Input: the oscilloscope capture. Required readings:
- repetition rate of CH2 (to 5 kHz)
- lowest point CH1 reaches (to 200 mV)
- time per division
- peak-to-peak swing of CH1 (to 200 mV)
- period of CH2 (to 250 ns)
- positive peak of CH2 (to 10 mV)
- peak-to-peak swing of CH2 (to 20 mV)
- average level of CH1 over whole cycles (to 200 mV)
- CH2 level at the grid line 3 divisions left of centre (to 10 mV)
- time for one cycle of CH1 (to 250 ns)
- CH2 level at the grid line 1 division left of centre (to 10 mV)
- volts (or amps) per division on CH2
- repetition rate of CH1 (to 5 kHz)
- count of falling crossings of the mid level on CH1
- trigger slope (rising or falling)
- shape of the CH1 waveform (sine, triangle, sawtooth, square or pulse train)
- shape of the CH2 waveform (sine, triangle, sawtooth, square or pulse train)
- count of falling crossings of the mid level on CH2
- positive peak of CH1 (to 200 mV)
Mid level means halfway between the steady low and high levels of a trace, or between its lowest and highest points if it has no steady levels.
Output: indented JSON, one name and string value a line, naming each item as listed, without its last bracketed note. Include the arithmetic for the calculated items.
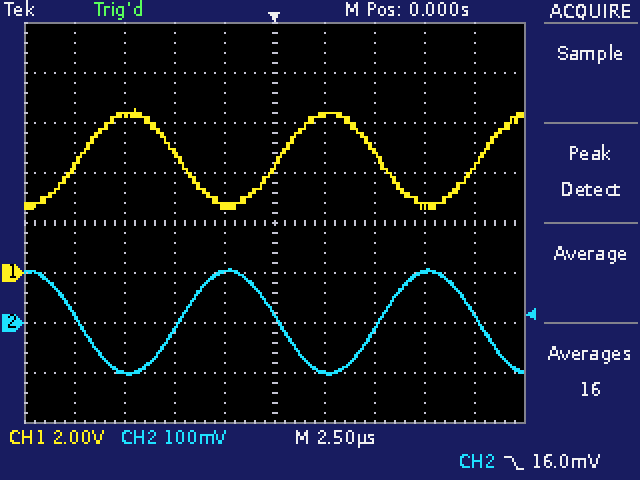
{
  "repetition rate of CH2": "1 / 10.00 µs ≈ 100 kHz",
  "lowest point CH1 reaches": "2.6 V",
  "time per division": "2.5 µs",
  "peak-to-peak swing of CH1": "6.6 V − (2.6 V) = 4.0 V",
  "period of CH2": "10.00 µs",
  "positive peak of CH2": "110 mV",
  "peak-to-peak swing of CH2": "220 mV",
  "average level of CH1 over whole cycles": "(6.6 V + (2.6 V)) / 2 ≈ 4.6 V",
  "CH2 level at the grid line 3 divisions left of centre": "-100 mV",
  "time for one cycle of CH1": "10.00 µs",
  "CH2 level at the grid line 1 division left of centre": "100 mV",
  "volts (or amps) per division on CH2": "100 mV",
  "repetition rate of CH1": "1 / 10.00 µs ≈ 100 kHz",
  "count of falling crossings of the mid level on CH1": "2",
  "trigger slope": "falling",
  "shape of the CH1 waveform": "sine",
  "shape of the CH2 waveform": "sine",
  "count of falling crossings of the mid level on CH2": "3",
  "positive peak of CH1": "6.6 V"
}
